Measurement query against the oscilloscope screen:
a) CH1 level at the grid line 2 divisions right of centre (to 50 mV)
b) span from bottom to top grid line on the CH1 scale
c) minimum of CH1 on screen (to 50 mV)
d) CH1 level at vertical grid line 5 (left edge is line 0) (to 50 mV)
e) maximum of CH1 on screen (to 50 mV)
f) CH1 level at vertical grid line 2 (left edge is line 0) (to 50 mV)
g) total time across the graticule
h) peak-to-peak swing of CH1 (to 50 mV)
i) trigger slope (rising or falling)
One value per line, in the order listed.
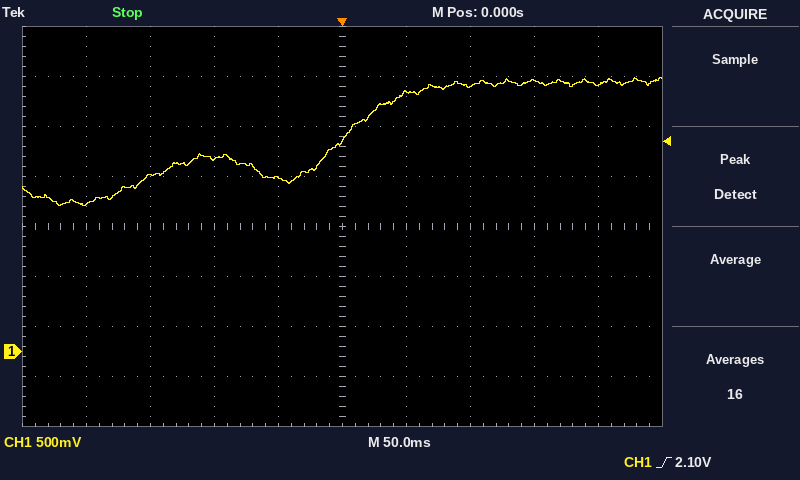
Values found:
2.65 V
4 V
1.45 V
2.10 V
2.75 V
1.75 V
500 ms
1.30 V
rising
